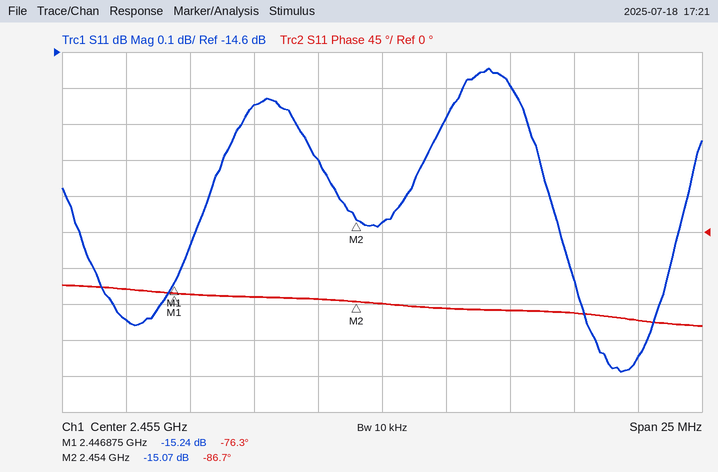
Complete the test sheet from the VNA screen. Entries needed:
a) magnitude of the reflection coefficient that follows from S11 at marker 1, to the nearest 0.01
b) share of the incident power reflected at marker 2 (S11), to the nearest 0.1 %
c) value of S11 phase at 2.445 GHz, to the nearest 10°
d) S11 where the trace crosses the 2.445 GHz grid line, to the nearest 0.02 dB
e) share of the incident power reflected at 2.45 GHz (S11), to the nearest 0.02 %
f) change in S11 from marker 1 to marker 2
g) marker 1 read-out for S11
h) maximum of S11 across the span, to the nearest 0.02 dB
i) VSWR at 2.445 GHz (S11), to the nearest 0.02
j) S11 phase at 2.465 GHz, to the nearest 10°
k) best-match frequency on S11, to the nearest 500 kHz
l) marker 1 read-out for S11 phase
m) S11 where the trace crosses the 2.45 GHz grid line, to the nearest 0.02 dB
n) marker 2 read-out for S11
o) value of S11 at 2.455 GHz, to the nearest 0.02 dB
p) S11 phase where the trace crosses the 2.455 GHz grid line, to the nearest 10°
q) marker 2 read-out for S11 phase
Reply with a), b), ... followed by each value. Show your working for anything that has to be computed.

a) 10^(-15.24/20) ≈ 0.17
b) 10^(-15.07/10) ≈ 3.1 %
c) -70°
d) -15.34 dB
e) 10^(-14.74/10) ≈ 3.36 %
f) -15.07 − (-15.24) = 0.17 dB
g) -15.24 dB
h) -14.64 dB
i) |Γ| = 10^(-15.34/20) = 0.1710; VSWR = (1 + 0.1710)/(1 − 0.1710) ≈ 1.41, so 1.42 to the nearest 0.02
j) -110°
k) 2.4645 GHz
l) -76.3°
m) -14.74 dB
n) -15.07 dB
o) -15.08 dB
p) -90°
q) -86.7°
